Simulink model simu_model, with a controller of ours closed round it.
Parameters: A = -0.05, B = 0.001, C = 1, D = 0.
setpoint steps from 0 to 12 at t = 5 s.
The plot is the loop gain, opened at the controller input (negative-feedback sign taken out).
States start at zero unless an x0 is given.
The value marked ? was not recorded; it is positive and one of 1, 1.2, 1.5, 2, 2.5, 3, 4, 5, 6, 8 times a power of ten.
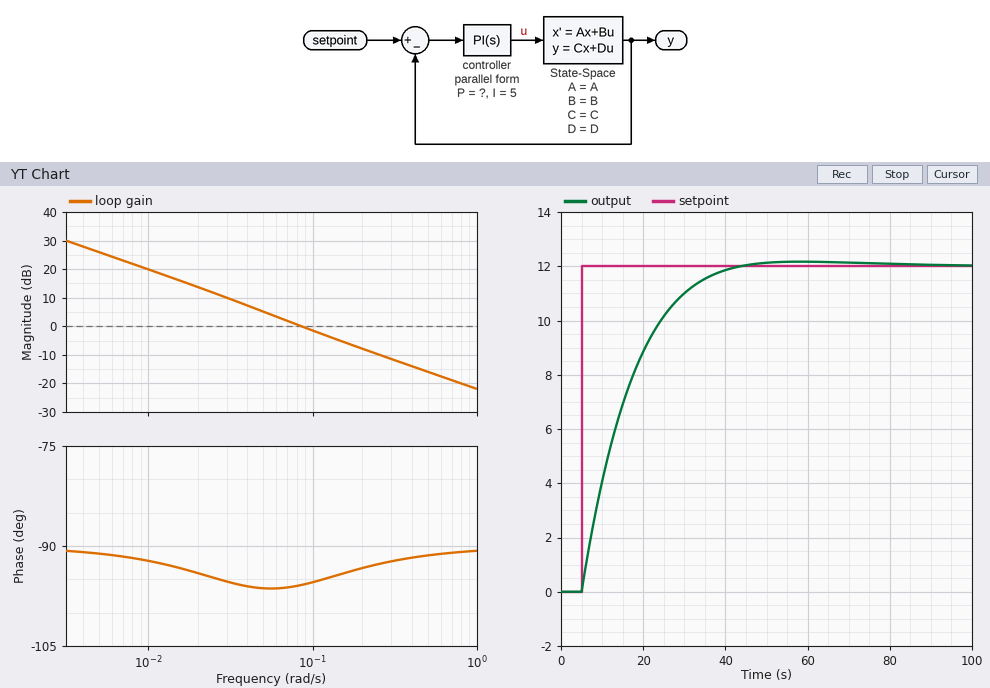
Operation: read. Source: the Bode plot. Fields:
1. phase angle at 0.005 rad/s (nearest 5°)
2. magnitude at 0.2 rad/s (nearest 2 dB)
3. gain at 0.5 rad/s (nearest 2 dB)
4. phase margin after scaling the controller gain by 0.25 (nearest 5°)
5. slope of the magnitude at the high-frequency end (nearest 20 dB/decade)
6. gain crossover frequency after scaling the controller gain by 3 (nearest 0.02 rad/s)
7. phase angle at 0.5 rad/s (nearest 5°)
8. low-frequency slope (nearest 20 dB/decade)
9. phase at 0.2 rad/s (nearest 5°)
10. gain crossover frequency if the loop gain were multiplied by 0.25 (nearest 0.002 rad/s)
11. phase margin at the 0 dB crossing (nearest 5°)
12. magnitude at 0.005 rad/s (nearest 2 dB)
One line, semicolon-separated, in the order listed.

-90°; -8 dB; -16 dB; 85°; -20 dB/decade; 0.24 rad/s; -90°; -20 dB/decade; -95°; 0.024 rad/s; 85°; 26 dB
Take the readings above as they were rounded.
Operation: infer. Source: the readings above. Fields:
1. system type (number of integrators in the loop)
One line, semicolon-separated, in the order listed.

1
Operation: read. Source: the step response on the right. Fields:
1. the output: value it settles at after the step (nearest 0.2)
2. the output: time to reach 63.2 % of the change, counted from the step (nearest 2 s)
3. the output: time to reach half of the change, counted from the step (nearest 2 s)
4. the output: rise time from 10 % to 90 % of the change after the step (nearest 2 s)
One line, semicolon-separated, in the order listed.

12.0; 12 s; 8 s; 22 s
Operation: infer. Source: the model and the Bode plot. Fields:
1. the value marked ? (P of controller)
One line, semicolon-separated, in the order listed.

80
